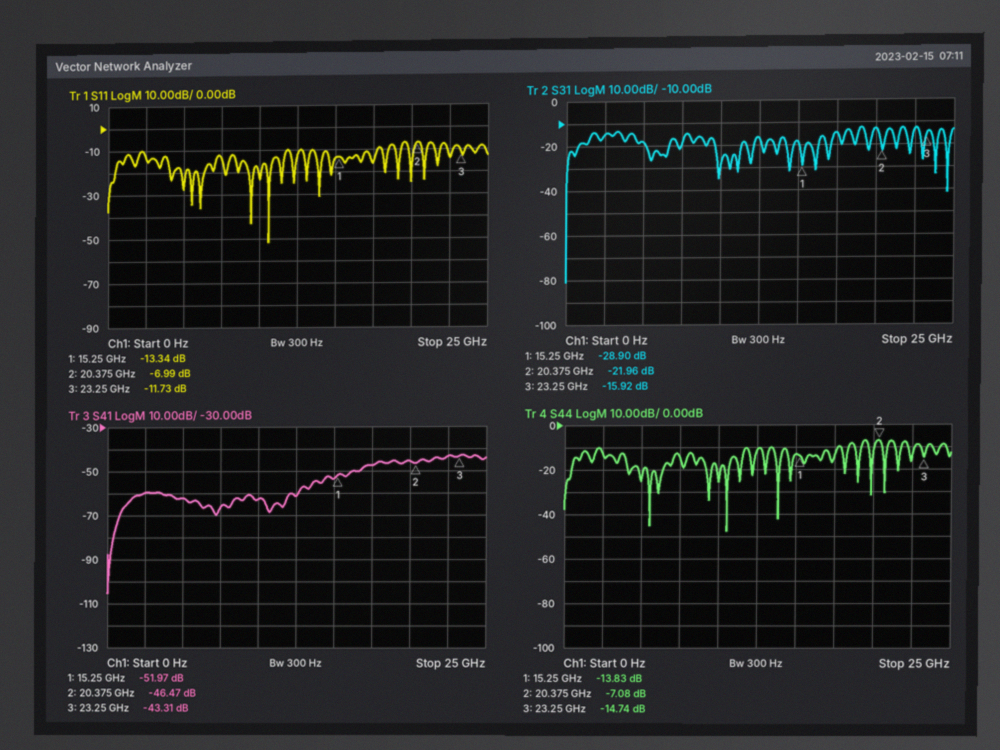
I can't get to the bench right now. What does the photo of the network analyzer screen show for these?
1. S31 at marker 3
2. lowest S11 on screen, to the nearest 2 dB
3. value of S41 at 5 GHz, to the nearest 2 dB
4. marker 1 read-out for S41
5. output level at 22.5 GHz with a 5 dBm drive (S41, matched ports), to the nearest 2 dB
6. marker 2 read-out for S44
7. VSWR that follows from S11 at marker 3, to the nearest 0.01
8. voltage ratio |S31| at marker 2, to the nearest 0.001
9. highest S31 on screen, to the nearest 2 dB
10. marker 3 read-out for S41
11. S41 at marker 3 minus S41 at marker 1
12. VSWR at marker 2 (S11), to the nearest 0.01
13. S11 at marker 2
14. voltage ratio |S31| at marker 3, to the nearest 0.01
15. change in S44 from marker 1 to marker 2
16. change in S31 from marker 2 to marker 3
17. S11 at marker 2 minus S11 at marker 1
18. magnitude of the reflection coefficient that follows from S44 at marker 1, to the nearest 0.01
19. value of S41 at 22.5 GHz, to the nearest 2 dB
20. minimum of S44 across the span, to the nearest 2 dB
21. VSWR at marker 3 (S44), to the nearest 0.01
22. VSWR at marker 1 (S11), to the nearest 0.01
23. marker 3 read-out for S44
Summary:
-15.92 dB
-52 dB
-62 dB
-51.97 dB
-38 dBm
-7.08 dB
1.70
0.080
-12 dB
-43.31 dB
8.66 dB
2.62
-6.99 dB
0.16
6.75 dB
6.04 dB
6.35 dB
0.20
-44 dB
-48 dB
1.45
1.55
-14.74 dB
